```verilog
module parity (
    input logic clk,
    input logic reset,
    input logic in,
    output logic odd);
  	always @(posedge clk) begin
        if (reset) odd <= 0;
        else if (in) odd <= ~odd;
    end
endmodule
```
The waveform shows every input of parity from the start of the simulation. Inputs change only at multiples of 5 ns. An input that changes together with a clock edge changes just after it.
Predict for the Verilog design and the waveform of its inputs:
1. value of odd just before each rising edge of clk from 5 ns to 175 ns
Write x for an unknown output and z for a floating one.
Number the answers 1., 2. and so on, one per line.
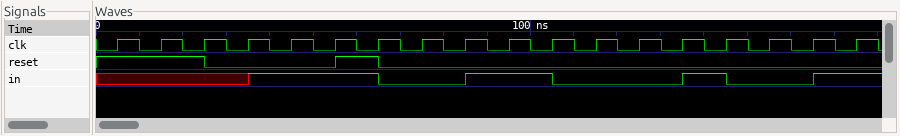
1. x 0 0 0 0 1 0 0 0 0 1 0 0 0 0 1 1 1
